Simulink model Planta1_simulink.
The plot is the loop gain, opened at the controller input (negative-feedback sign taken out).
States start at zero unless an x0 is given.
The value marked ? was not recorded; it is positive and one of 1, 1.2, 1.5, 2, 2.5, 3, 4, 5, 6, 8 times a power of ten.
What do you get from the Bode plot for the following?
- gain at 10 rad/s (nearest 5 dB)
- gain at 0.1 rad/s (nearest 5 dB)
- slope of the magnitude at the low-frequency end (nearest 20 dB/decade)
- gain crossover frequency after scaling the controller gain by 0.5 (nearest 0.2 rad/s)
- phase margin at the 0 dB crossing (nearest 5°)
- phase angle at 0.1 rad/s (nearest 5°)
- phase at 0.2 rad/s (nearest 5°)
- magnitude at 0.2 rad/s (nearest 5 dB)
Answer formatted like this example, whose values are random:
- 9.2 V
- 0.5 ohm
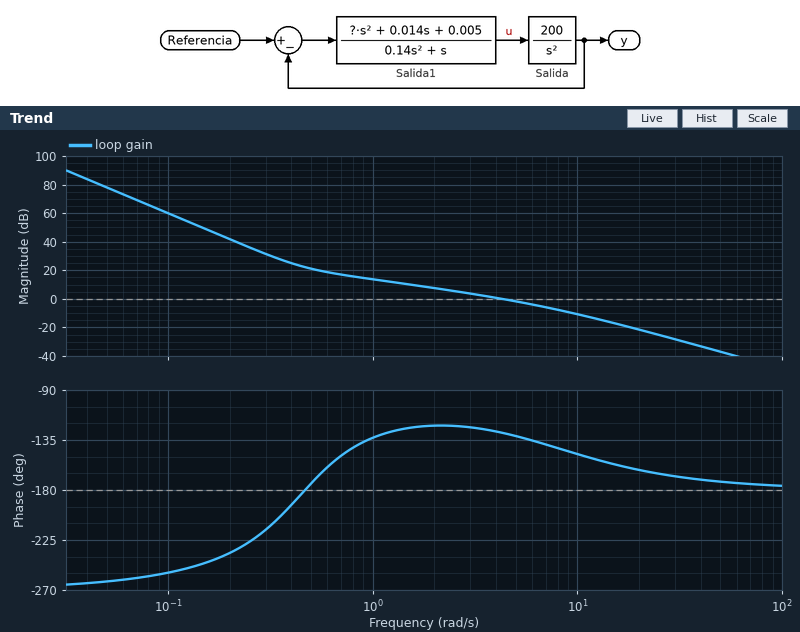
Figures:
- -10 dB
- 60 dB
- -60 dB/decade
- 2.4 rad/s
- 50°
- -255°
- -235°
- 40 dB
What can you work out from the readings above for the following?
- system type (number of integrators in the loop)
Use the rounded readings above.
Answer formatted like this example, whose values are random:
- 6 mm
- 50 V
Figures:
- 3
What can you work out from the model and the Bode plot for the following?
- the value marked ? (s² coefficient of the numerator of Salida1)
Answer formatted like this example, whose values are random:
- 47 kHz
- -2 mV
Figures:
- 0.025
